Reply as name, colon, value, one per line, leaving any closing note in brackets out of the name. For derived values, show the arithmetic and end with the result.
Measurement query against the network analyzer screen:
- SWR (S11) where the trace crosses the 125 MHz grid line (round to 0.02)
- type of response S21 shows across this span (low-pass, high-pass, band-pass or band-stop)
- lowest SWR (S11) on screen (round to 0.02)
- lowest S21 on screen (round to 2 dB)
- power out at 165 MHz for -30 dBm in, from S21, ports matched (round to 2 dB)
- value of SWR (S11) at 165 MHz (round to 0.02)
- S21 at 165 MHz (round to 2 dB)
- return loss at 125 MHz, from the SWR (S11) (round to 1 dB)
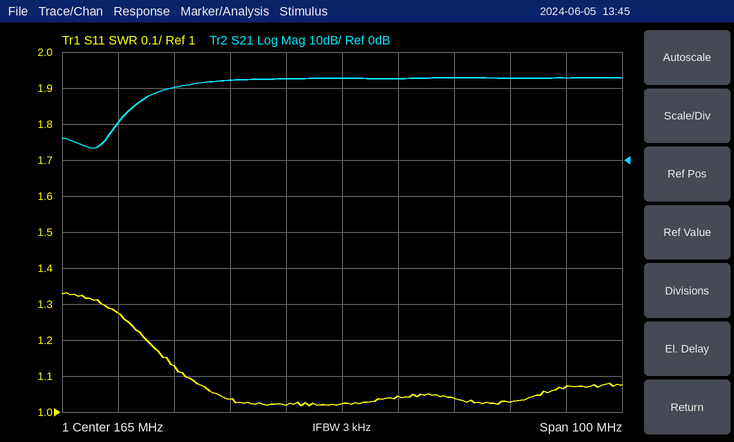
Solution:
SWR (S11) where the trace crosses the 125 MHz grid line: 1.28
type of response S21 shows across this span: high-pass
lowest SWR (S11) on screen: 1.02
lowest S21 on screen: 4 dB
power out at 165 MHz for -30 dBm in, from S21, ports matched: -30 dBm + (22 dB) = -8 dBm
value of SWR (S11) at 165 MHz: 1.02
S21 at 165 MHz: 22 dB
return loss at 125 MHz, from the SWR (S11): −20 log10((1.28 − 1)/(1.28 + 1)) ≈ 18 dB
